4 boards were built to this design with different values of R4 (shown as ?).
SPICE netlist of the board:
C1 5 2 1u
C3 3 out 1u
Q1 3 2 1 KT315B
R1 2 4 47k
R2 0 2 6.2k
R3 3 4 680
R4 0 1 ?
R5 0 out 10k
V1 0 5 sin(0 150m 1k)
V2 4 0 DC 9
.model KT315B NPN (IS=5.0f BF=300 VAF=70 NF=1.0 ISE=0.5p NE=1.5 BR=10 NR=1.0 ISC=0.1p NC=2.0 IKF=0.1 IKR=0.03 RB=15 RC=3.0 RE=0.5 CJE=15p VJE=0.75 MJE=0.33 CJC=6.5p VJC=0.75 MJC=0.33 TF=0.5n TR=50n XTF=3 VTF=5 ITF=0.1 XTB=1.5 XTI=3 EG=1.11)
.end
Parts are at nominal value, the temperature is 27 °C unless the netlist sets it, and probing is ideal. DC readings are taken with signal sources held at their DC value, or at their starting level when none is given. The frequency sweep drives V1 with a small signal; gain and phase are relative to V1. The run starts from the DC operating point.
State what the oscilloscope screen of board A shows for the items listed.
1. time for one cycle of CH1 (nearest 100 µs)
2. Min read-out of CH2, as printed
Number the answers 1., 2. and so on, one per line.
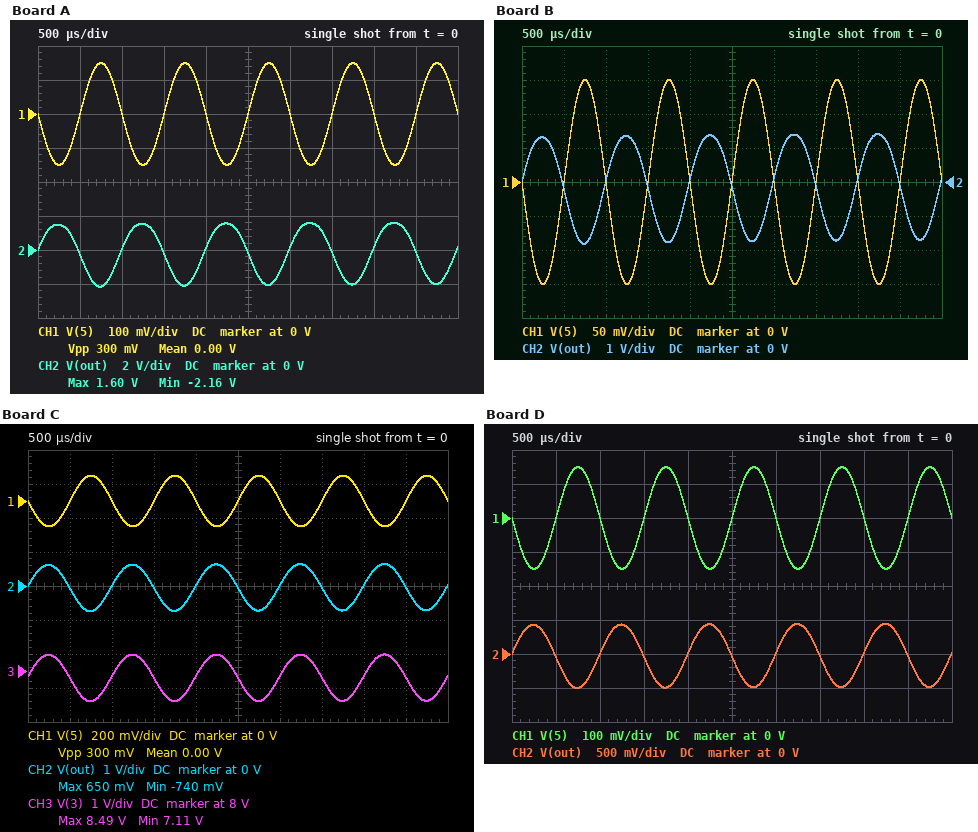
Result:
1. 1.0 ms
2. -2.16 V
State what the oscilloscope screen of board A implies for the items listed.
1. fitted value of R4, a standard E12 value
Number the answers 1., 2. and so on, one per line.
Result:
1. 39 Ω
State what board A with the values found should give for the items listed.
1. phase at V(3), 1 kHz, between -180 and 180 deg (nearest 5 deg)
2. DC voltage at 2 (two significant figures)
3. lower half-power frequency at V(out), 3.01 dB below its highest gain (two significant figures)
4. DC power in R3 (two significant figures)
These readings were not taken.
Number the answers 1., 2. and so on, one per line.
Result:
1. 5 deg
2. 820 mV
3. 69 Hz
4. 5.7 mW
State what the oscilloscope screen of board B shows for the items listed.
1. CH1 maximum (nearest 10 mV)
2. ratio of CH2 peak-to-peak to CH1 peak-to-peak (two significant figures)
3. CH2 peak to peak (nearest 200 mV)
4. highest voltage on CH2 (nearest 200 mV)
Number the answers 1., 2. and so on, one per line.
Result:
1. 150 mV
2. 11
3. 3.2 V
4. 1.4 V
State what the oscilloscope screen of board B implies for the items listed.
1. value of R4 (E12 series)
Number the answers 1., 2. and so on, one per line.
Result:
1. 47 Ω
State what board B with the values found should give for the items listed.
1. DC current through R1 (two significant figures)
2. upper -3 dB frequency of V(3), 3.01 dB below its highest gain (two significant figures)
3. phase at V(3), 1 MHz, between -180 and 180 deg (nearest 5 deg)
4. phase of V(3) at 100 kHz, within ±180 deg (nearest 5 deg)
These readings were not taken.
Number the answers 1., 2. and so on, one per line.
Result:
1. 170 µA
2. 57 MHz
3. 0 deg
4. 0 deg
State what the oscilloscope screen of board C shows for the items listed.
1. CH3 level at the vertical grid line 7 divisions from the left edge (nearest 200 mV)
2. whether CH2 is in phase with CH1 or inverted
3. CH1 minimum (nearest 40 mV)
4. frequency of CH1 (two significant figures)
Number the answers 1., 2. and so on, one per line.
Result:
1. 7.8 V
2. inverted
3. -160 mV
4. 1.0 kHz
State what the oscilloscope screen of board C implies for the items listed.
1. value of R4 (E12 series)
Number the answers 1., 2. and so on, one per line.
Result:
1. 120 Ω
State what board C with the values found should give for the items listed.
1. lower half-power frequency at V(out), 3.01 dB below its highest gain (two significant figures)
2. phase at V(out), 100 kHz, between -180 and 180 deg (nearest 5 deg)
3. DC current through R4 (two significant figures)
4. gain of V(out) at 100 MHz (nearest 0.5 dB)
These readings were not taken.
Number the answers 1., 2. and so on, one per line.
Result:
1. 48 Hz
2. 0 deg
3. 1.7 mA
4. 9.0 dB
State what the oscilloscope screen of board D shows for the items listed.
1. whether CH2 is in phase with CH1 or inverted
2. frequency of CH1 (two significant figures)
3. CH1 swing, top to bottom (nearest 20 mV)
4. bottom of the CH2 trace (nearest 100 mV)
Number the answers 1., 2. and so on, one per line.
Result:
1. inverted
2. 1.0 kHz
3. 300 mV
4. -500 mV
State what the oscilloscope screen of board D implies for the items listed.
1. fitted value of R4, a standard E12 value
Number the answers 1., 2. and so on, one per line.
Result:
1. 180 Ω
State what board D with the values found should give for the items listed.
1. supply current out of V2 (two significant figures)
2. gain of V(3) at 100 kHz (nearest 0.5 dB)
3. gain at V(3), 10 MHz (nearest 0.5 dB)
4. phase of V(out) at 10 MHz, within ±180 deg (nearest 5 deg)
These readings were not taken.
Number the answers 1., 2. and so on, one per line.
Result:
1. 1.5 mA
2. 10.0 dB
3. 10.0 dB
4. -15 deg
